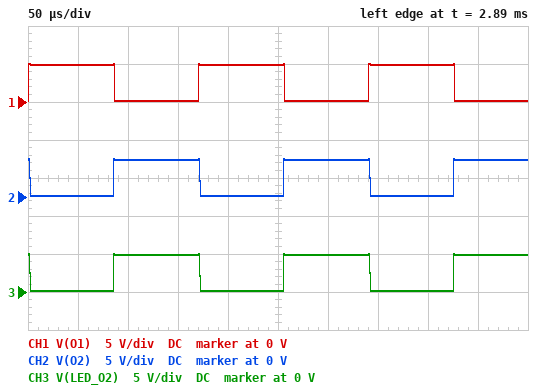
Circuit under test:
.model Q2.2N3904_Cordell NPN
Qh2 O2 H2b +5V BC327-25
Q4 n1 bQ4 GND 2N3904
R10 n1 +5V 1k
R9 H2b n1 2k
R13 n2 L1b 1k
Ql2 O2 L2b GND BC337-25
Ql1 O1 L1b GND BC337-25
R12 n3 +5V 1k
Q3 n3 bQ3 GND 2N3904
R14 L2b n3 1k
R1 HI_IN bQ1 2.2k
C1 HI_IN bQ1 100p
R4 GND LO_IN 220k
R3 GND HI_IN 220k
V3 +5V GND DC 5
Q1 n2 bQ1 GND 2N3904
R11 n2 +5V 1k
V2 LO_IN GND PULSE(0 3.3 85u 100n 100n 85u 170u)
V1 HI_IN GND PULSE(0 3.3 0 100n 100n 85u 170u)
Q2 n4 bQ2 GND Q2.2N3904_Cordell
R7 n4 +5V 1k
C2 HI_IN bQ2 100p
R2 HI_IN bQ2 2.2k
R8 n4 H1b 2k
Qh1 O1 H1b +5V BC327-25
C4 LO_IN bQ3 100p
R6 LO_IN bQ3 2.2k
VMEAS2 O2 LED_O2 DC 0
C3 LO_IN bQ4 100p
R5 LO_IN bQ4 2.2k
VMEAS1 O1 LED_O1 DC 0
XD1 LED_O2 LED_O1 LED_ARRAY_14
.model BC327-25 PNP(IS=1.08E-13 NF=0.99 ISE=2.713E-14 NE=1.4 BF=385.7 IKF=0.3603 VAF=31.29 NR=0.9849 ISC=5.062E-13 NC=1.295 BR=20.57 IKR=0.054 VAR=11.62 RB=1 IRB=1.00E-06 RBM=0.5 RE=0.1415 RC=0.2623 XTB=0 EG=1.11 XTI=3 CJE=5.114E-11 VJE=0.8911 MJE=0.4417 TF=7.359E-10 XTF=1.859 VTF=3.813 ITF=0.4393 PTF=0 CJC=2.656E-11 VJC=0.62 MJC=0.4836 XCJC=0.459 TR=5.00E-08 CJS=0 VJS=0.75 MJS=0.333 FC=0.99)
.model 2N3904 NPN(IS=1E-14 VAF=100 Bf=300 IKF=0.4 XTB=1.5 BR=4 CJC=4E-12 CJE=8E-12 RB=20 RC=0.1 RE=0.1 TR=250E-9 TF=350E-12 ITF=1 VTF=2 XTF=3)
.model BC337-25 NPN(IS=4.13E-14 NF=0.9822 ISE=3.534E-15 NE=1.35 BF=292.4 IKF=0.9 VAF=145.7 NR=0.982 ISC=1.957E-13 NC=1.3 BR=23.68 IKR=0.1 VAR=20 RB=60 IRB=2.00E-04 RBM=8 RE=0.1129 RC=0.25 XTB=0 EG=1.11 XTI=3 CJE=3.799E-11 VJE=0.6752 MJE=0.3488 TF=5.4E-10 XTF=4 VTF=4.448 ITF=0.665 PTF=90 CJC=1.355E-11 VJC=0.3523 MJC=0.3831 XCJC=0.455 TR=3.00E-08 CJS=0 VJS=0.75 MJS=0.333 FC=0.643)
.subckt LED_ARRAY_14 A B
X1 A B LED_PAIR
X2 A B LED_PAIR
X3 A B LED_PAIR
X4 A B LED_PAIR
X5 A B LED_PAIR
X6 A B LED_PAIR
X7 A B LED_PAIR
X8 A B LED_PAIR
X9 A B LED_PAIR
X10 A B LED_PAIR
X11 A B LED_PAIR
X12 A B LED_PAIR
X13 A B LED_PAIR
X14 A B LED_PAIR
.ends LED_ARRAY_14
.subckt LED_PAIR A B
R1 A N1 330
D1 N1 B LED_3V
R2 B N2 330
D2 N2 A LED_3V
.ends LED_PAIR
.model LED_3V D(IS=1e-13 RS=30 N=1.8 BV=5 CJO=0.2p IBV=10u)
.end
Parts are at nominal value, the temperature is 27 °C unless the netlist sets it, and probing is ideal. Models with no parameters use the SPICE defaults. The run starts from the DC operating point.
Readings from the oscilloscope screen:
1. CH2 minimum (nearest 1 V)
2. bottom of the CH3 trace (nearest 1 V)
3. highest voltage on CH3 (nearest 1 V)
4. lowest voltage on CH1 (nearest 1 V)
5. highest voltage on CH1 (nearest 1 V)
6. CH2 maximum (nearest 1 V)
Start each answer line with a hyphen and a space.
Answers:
- 0 V
- 0 V
- 5 V
- 0 V
- 5 V
- 5 V
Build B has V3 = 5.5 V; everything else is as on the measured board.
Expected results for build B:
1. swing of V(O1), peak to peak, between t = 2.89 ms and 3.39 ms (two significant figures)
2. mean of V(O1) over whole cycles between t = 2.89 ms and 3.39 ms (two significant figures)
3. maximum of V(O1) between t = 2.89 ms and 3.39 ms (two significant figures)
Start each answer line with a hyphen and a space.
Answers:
- 5.4 V
- 2.8 V
- 5.5 V
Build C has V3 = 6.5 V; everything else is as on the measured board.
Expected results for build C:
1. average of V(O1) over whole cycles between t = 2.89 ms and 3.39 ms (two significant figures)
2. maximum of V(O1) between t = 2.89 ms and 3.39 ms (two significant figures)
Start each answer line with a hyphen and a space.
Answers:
- 3.3 V
- 6.5 V
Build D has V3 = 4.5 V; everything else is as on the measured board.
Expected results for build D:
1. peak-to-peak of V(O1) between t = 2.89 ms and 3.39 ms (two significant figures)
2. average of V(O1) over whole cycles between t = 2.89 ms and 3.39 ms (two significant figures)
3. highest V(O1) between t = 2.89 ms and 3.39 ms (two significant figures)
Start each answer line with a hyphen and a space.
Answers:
- 4.4 V
- 2.3 V
- 4.5 V
